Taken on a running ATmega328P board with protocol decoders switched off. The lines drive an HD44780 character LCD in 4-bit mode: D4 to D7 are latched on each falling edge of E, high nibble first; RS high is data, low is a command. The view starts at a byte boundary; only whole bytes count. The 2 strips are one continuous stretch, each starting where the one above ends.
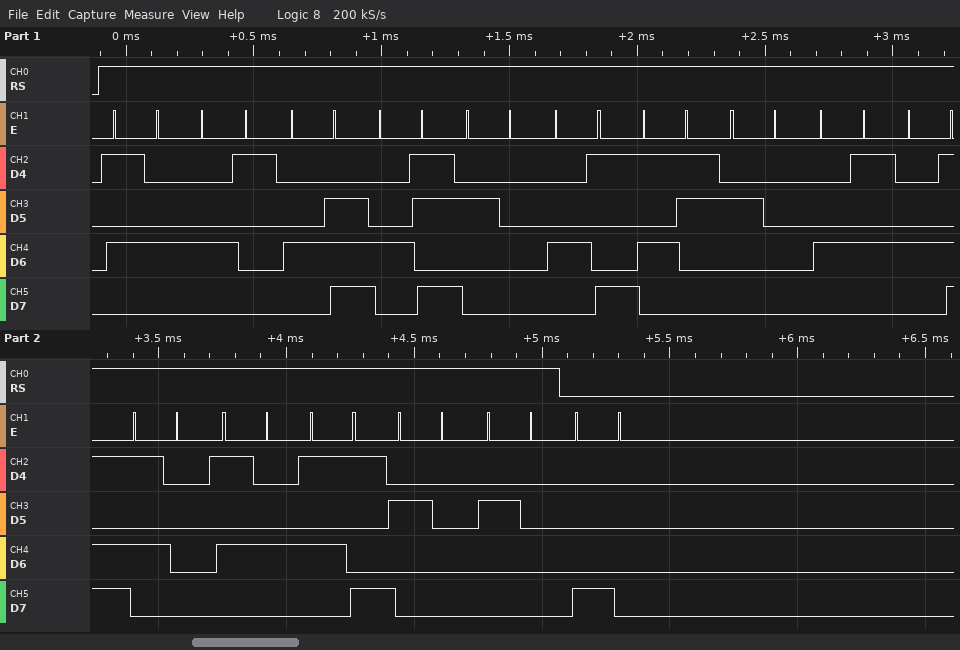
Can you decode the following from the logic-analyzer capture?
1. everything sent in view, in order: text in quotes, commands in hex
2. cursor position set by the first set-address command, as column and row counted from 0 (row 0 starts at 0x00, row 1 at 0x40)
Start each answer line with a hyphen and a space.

- "TANK IS EMPTY  " 0x80
- column 0, row 0
